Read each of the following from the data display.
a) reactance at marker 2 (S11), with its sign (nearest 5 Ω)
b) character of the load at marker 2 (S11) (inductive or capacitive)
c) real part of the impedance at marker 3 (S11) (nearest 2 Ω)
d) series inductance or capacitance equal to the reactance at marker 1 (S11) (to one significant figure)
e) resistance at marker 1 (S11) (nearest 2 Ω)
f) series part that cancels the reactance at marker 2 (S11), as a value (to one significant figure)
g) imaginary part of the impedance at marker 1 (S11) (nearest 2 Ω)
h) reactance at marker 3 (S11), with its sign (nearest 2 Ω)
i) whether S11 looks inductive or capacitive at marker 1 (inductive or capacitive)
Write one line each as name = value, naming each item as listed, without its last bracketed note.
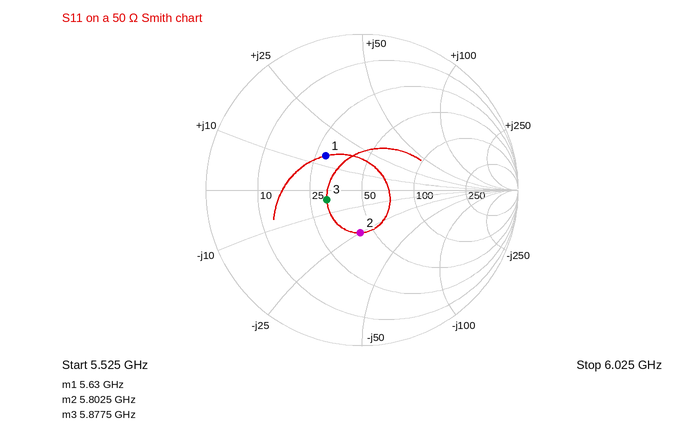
reactance at marker 2 (S11), with its sign = -25 Ω
character of the load at marker 2 (S11) = capacitive
real part of the impedance at marker 3 (S11) = 32 Ω
series inductance or capacitance equal to the reactance at marker 1 (S11) = 400 pH
resistance at marker 1 (S11) = 28 Ω
series part that cancels the reactance at marker 2 (S11), as a value = 700 pH
imaginary part of the impedance at marker 1 (S11) = +14 Ω
reactance at marker 3 (S11), with its sign = -4 Ω
whether S11 looks inductive or capacitive at marker 1 = inductive
